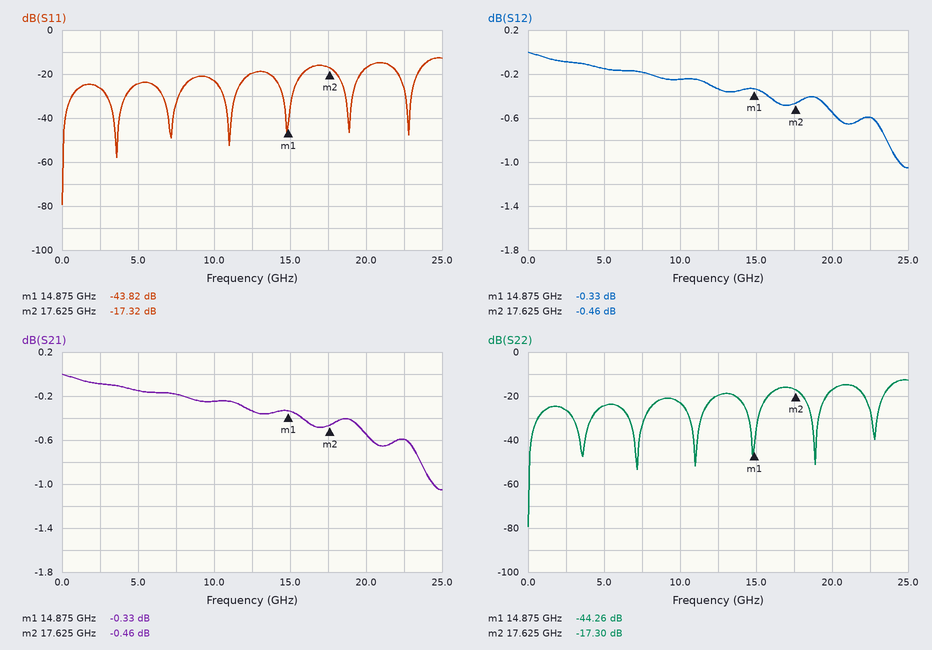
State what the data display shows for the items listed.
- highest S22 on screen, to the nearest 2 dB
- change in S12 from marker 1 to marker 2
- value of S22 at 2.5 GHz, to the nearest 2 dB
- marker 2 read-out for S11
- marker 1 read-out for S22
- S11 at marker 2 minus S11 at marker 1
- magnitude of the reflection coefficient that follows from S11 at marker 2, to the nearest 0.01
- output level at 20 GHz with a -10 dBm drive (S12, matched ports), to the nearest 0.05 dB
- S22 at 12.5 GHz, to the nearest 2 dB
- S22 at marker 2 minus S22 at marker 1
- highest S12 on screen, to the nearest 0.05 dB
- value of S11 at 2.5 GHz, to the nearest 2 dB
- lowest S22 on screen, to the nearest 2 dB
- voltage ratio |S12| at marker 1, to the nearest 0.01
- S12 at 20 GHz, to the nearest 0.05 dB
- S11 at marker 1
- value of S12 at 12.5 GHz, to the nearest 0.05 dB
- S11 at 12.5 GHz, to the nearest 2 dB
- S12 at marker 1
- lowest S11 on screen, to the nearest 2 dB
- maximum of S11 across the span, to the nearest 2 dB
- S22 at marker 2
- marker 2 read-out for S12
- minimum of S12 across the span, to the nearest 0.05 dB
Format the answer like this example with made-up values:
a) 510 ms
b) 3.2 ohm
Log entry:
a) -12 dB
b) -0.13 dB
c) -26 dB
d) -17.32 dB
e) -44.26 dB
f) 26.50 dB
g) 0.14
h) -10.55 dBm
i) -20 dB
j) 26.96 dB
k) 0.00 dB
l) -26 dB
m) -80 dB
n) 0.96
o) -0.55 dB
p) -43.82 dB
q) -0.35 dB
r) -20 dB
s) -0.33 dB
t) -80 dB
u) -12 dB
v) -17.30 dB
w) -0.46 dB
x) -1.05 dB
